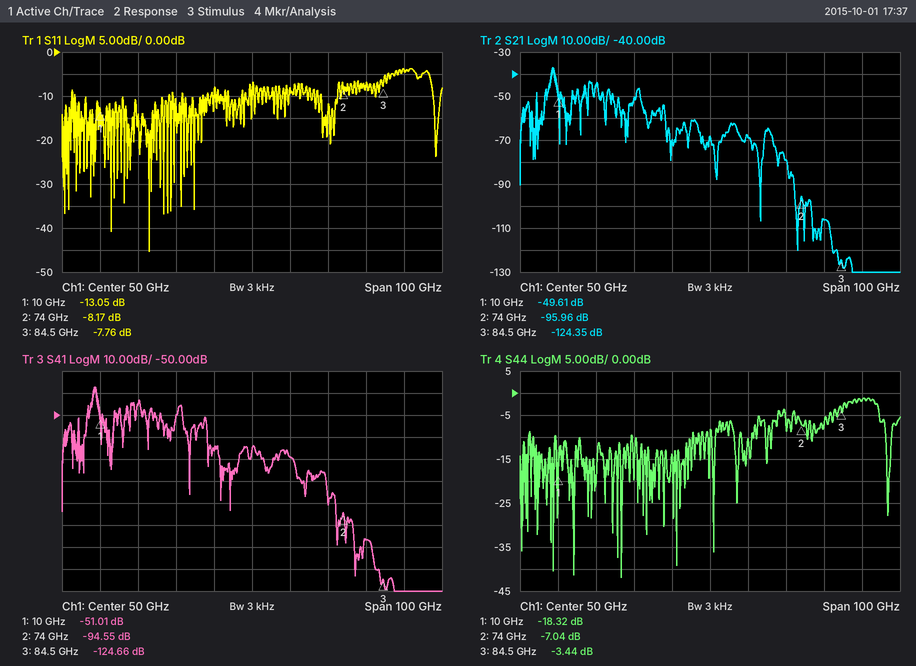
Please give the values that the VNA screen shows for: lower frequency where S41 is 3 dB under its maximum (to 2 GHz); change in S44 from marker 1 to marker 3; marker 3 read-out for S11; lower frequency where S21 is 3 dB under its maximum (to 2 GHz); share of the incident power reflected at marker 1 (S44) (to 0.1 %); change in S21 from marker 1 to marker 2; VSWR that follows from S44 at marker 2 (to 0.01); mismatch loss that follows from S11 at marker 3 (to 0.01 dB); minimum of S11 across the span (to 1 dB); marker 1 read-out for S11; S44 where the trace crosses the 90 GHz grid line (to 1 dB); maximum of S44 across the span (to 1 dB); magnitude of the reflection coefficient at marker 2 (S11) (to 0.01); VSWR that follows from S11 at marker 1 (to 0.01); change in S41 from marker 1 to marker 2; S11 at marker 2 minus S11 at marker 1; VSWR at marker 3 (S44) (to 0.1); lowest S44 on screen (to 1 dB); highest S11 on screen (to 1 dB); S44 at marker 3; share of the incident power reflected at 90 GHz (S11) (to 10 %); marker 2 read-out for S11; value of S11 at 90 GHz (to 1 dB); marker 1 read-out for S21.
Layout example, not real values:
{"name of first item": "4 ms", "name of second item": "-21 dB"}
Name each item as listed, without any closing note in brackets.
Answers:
{"lower frequency where S41 is 3 dB under its maximum": "8 GHz", "change in S44 from marker 1 to marker 3": "14.88 dB", "marker 3 read-out for S11": "-7.76 dB", "lower frequency where S21 is 3 dB under its maximum": "8 GHz", "share of the incident power reflected at marker 1 (S44)": "1.5 %", "change in S21 from marker 1 to marker 2": "-46.35 dB", "VSWR that follows from S44 at marker 2": "2.60", "mismatch loss that follows from S11 at marker 3": "0.80 dB", "minimum of S11 across the span": "-45 dB", "marker 1 read-out for S11": "-13.05 dB", "S44 where the trace crosses the 90 GHz grid line": "-2 dB", "maximum of S44 across the span": "-1 dB", "magnitude of the reflection coefficient at marker 2 (S11)": "0.39", "VSWR that follows from S11 at marker 1": "1.57", "change in S41 from marker 1 to marker 2": "-43.54 dB", "S11 at marker 2 minus S11 at marker 1": "4.88 dB", "VSWR at marker 3 (S44)": "5.1", "lowest S44 on screen": "-42 dB", "highest S11 on screen": "-4 dB", "S44 at marker 3": "-3.44 dB", "share of the incident power reflected at 90 GHz (S11)": "40 %", "marker 2 read-out for S11": "-8.17 dB", "value of S11 at 90 GHz": "-4 dB", "marker 1 read-out for S21": "-49.61 dB"}
